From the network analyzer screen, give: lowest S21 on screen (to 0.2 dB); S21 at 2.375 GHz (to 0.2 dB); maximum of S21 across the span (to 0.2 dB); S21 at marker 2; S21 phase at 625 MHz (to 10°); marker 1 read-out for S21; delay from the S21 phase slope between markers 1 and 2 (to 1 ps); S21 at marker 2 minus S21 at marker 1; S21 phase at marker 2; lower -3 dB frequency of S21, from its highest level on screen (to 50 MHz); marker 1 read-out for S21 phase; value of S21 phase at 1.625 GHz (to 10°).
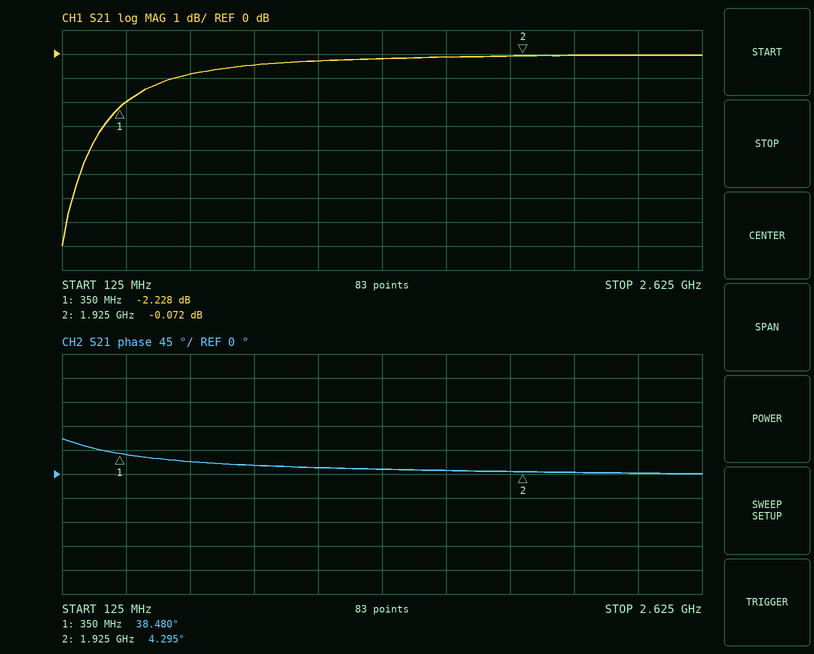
-8.0 dB
0.0 dB
0.0 dB
-0.072 dB
20°
-2.228 dB
60 ps
2.156 dB
4.295°
300 MHz
38.480°
10°
